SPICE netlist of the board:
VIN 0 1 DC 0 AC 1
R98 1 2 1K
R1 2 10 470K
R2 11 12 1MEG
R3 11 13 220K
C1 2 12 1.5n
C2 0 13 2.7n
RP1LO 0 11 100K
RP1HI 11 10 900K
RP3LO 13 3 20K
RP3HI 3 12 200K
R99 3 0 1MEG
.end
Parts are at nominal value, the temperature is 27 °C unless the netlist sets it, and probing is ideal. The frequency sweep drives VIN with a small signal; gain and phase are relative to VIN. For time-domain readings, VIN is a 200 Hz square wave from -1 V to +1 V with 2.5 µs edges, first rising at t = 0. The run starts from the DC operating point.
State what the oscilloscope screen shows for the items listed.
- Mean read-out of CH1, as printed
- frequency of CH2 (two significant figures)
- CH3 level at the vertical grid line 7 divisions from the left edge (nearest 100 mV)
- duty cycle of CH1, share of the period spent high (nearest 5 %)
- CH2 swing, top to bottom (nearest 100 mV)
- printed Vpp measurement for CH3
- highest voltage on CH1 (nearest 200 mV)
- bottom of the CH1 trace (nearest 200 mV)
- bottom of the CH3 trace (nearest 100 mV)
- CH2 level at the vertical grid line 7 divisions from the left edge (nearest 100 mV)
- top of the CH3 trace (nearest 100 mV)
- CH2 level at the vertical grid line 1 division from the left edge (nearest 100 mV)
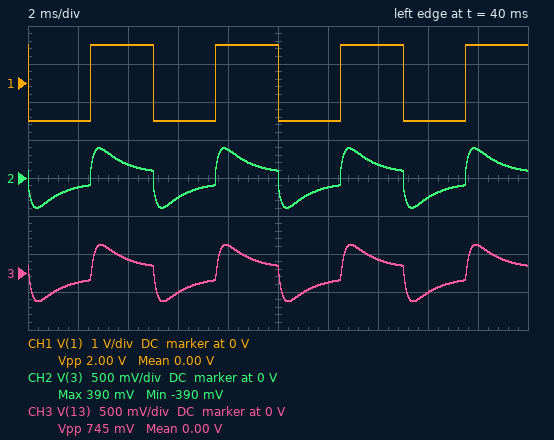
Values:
0.00 V
200 Hz
200 mV
50 %
800 mV
745 mV
1.0 V
-1.0 V
-400 mV
200 mV
400 mV
-100 mV
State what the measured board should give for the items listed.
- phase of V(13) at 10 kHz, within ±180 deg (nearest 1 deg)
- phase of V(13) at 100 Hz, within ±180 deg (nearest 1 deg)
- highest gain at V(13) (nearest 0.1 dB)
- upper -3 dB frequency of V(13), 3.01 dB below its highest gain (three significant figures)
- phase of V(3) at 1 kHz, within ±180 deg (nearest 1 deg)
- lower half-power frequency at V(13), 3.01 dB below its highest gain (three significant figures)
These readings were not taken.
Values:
96 deg
-143 deg
-11.5 dB
1.21 kHz
157 deg
123 Hz
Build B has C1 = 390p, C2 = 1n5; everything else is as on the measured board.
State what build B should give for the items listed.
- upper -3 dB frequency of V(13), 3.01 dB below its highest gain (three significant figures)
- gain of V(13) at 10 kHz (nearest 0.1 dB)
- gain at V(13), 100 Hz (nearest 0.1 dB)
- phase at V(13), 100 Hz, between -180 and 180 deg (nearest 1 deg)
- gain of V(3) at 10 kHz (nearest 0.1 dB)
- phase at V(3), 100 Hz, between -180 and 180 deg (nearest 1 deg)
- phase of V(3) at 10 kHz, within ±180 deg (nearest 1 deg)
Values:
3.42 kHz
-26.0 dB
-23.1 dB
-154 deg
-20.0 dB
-152 deg
166 deg
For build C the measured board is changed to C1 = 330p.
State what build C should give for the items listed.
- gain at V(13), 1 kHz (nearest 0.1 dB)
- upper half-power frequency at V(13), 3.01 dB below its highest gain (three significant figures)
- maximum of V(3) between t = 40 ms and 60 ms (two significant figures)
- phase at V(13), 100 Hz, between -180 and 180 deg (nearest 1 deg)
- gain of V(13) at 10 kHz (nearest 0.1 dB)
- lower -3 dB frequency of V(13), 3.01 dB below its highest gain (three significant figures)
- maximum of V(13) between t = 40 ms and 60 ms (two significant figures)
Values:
-20.7 dB
3.28 kHz
130 mV
-167 deg
-31.1 dB
126 Hz
120 mV
